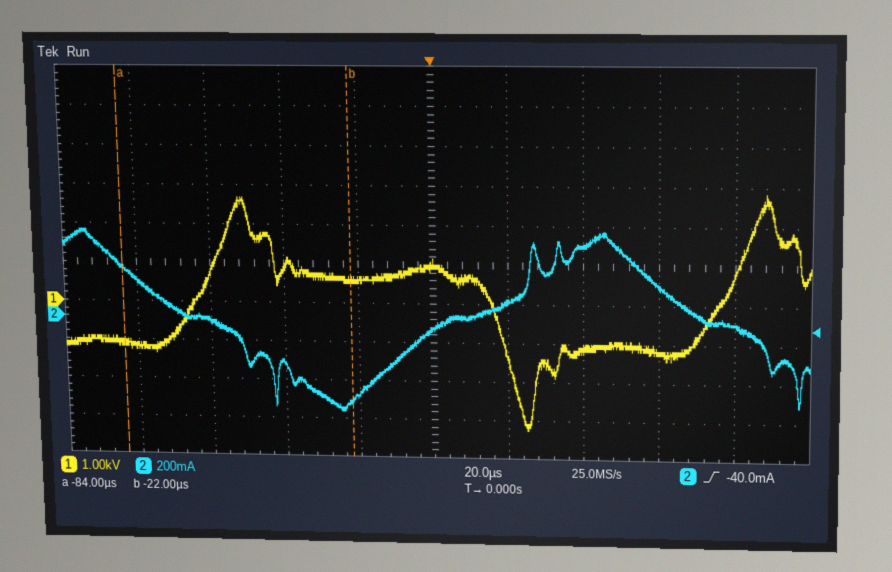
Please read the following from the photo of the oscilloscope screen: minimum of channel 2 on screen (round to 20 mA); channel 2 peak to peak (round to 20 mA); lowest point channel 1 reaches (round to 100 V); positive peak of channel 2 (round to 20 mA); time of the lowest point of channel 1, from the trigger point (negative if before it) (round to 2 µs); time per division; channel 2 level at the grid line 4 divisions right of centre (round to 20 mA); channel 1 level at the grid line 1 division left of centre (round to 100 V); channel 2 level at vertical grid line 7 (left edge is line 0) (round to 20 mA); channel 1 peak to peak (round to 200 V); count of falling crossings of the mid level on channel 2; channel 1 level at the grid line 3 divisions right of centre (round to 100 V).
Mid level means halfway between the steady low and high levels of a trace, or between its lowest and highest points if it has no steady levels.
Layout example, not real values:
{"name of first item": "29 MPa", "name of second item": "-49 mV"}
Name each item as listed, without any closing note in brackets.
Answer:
{"minimum of channel 2 on screen": "-480 mA", "channel 2 peak to peak": "940 mA", "lowest point channel 1 reaches": "-3.2 kV", "positive peak of channel 2": "460 mA", "time of the lowest point of channel 1, from the trigger point (negative if before it)": "+26 µs", "time per division": "20 µs", "channel 2 level at the grid line 4 divisions right of centre": "-20 mA", "channel 1 level at the grid line 1 division left of centre": "600 V", "channel 2 level at vertical grid line 7 (left edge is line 0)": "380 mA", "channel 1 peak to peak": "6.0 kV", "count of falling crossings of the mid level on channel 2": "2", "channel 1 level at the grid line 3 divisions right of centre": "-1.2 kV"}
